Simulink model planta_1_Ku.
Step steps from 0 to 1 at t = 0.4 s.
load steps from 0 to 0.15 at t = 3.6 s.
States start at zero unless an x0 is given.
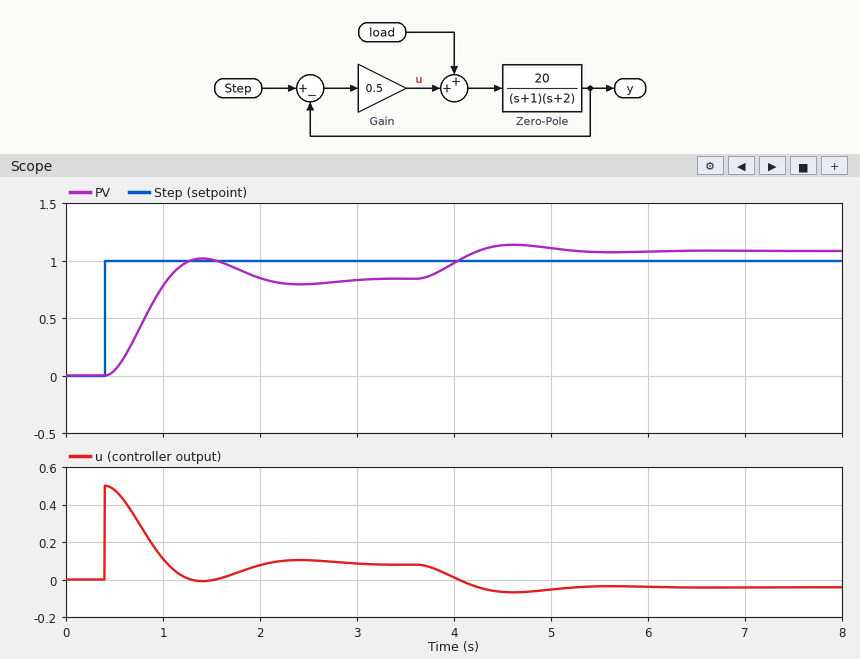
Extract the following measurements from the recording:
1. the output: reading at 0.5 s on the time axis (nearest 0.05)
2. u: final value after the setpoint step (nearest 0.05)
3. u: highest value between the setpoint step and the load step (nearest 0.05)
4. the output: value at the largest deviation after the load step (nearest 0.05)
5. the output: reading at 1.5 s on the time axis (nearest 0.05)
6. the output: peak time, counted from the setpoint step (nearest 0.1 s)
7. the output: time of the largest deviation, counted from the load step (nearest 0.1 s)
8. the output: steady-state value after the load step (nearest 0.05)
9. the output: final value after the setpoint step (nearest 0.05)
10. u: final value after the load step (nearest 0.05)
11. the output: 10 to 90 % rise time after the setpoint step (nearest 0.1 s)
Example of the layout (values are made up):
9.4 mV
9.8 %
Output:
0.05
0.10
0.50
1.15
1.00
1.0 s
1.0 s
1.10
0.85
-0.05
0.4 s
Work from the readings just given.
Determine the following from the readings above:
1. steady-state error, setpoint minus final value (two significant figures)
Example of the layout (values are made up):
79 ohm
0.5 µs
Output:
0.15
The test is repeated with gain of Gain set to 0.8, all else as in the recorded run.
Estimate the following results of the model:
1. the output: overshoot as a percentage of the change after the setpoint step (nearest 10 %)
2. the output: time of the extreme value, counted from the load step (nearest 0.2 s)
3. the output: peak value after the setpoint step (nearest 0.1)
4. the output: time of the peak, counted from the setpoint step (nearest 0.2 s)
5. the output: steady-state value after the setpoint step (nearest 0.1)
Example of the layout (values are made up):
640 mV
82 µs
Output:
30 %
0.8 s
1.2
0.8 s
0.9
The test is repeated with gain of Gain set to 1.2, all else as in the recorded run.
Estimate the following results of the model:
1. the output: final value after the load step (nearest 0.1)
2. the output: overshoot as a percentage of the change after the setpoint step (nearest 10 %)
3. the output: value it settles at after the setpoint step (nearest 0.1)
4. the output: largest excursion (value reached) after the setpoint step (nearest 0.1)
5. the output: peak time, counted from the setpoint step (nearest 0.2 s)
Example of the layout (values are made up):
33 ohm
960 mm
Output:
1.0
40 %
0.9
1.3
0.6 s
